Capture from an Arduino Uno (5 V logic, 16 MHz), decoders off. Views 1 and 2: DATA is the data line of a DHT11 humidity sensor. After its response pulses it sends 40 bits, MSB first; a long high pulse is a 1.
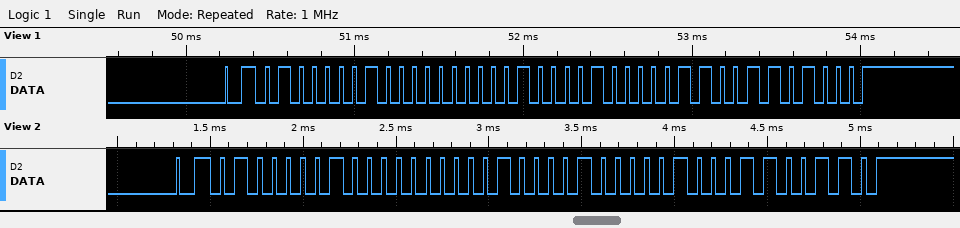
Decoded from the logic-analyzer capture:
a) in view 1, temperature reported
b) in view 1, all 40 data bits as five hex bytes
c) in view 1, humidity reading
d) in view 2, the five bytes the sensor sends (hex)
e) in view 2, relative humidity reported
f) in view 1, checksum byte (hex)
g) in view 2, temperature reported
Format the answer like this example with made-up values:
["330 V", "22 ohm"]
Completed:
["33.6 °C", "41 00 21 06 68", "65 %", "41 00 21 04 66", "65 %", "0x68", "33.4 °C"]
